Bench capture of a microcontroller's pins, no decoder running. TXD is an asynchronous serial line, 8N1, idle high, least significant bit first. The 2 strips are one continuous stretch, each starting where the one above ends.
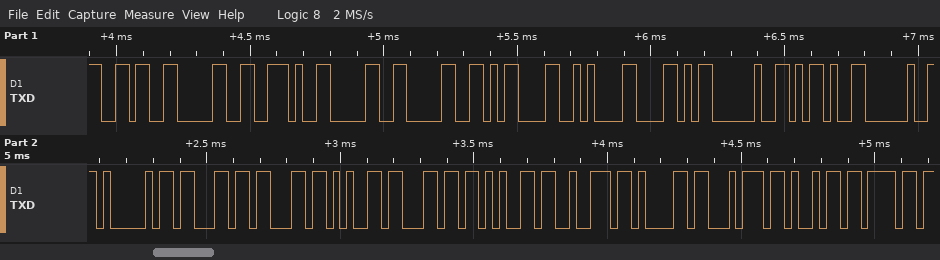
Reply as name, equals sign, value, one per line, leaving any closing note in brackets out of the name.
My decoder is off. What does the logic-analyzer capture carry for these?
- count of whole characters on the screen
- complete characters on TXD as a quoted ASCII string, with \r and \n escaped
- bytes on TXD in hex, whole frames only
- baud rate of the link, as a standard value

count of whole characters on the screen = 22
complete characters on TXD as a quoted ASCII string, with \r and \n escaped = "60.00\r\nX - Acceleratio"
bytes on TXD in hex, whole frames only = 36 30 2E 30 30 0D 0A 58 20 2D 20 41 63 63 65 6C 65 72 61 74 69 6F
baud rate of the link, as a standard value = 38400 baud
